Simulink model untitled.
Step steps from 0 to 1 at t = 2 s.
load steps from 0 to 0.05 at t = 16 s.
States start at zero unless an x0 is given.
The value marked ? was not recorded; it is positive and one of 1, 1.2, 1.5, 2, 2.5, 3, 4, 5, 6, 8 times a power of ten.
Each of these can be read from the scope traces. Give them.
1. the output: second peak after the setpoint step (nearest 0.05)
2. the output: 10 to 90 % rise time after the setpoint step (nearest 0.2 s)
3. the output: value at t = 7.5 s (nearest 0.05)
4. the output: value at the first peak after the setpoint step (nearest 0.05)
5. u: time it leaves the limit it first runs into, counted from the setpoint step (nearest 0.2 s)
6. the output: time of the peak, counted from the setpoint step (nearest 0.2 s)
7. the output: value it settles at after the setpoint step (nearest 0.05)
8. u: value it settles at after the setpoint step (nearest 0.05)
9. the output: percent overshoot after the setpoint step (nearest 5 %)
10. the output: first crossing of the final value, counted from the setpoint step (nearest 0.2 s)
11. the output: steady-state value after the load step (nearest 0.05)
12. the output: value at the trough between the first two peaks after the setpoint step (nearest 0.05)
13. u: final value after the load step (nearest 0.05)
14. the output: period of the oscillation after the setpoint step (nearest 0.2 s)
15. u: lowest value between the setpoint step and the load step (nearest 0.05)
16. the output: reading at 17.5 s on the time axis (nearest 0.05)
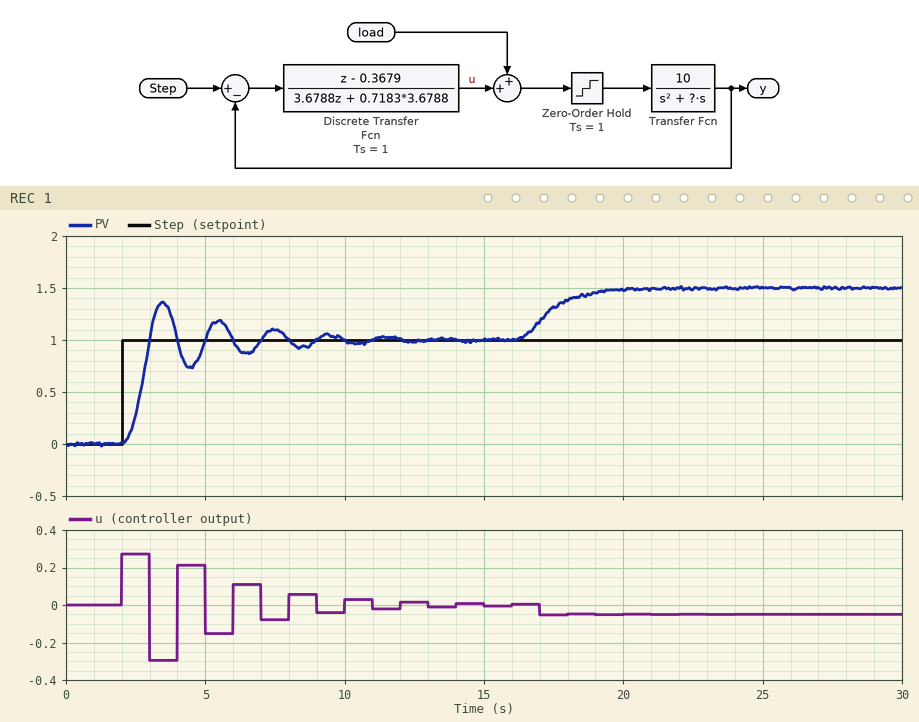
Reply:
1.20
0.6 s
1.10
1.35
1.0 s
1.4 s
1.00
0.00
35 %
1.0 s
1.50
0.75
-0.05
2.0 s
-0.30
1.30
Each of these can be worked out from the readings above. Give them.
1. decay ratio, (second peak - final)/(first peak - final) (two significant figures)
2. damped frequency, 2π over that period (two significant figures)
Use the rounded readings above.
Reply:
0.57
3.1 rad/s
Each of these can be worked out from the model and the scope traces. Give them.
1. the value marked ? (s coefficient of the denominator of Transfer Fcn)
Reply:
1
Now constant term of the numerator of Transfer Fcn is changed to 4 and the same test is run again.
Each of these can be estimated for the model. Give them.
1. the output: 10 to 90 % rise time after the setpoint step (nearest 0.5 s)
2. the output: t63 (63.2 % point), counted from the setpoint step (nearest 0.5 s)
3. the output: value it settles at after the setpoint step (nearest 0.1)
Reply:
4.5 s
1.5 s
1.0
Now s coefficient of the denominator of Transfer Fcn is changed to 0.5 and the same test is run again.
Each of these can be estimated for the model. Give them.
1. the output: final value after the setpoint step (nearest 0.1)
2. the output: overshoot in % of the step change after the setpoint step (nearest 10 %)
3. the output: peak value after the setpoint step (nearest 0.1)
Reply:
1.0
70 %
1.7
